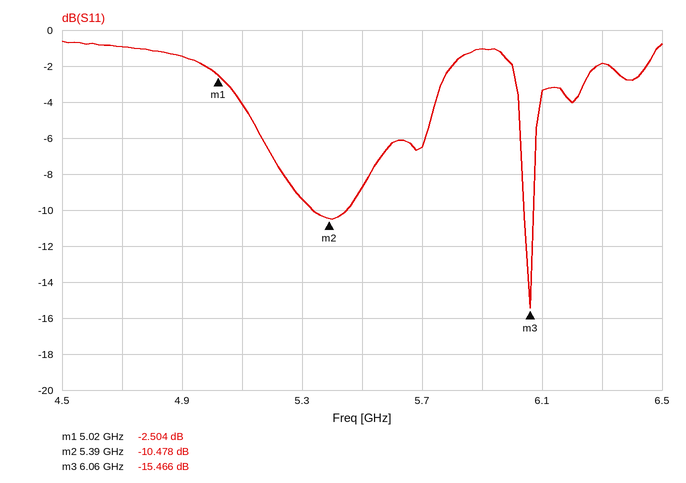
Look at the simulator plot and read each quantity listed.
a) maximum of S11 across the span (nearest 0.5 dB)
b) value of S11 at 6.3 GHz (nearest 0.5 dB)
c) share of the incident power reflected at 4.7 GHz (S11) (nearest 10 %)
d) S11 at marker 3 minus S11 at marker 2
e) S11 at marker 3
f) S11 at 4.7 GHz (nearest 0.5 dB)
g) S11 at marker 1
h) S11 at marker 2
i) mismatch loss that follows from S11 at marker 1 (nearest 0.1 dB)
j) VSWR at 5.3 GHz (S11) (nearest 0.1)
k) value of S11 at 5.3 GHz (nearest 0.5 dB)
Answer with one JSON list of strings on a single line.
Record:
["-0.5 dB", "-2.0 dB", "80 %", "-4.988 dB", "-15.466 dB", "-1.0 dB", "-2.504 dB", "-10.478 dB", "3.6 dB", "2.0", "-9.5 dB"]
